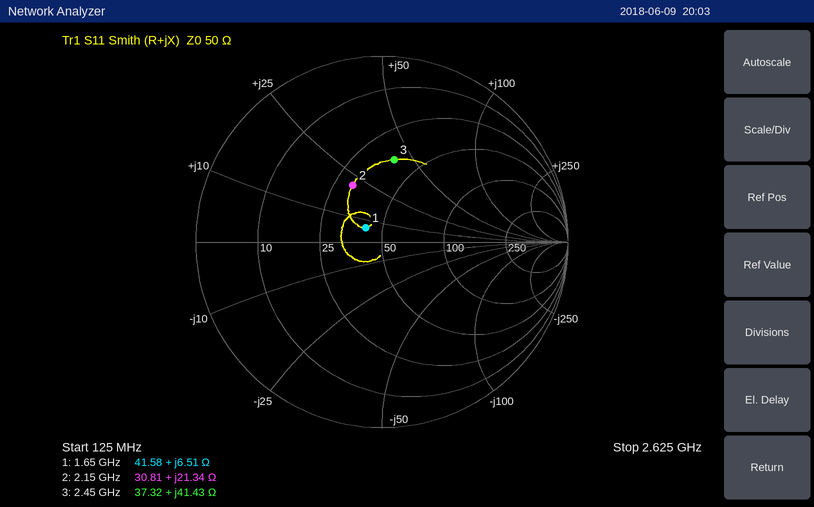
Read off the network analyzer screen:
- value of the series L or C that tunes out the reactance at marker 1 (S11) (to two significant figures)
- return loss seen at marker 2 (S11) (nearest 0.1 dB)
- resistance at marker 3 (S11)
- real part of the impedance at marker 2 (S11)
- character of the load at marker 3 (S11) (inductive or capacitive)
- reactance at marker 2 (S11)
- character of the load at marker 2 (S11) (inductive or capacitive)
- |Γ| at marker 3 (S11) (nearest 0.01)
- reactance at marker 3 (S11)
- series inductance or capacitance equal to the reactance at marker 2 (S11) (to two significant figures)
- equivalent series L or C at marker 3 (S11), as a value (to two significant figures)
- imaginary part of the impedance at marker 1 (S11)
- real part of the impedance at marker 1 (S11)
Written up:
15 pF
9.3 dB
37.32 Ω
30.81 Ω
inductive
+21.34 Ω
inductive
0.45
+41.43 Ω
1.6 nH
2.7 nH
+6.51 Ω
41.58 Ω
